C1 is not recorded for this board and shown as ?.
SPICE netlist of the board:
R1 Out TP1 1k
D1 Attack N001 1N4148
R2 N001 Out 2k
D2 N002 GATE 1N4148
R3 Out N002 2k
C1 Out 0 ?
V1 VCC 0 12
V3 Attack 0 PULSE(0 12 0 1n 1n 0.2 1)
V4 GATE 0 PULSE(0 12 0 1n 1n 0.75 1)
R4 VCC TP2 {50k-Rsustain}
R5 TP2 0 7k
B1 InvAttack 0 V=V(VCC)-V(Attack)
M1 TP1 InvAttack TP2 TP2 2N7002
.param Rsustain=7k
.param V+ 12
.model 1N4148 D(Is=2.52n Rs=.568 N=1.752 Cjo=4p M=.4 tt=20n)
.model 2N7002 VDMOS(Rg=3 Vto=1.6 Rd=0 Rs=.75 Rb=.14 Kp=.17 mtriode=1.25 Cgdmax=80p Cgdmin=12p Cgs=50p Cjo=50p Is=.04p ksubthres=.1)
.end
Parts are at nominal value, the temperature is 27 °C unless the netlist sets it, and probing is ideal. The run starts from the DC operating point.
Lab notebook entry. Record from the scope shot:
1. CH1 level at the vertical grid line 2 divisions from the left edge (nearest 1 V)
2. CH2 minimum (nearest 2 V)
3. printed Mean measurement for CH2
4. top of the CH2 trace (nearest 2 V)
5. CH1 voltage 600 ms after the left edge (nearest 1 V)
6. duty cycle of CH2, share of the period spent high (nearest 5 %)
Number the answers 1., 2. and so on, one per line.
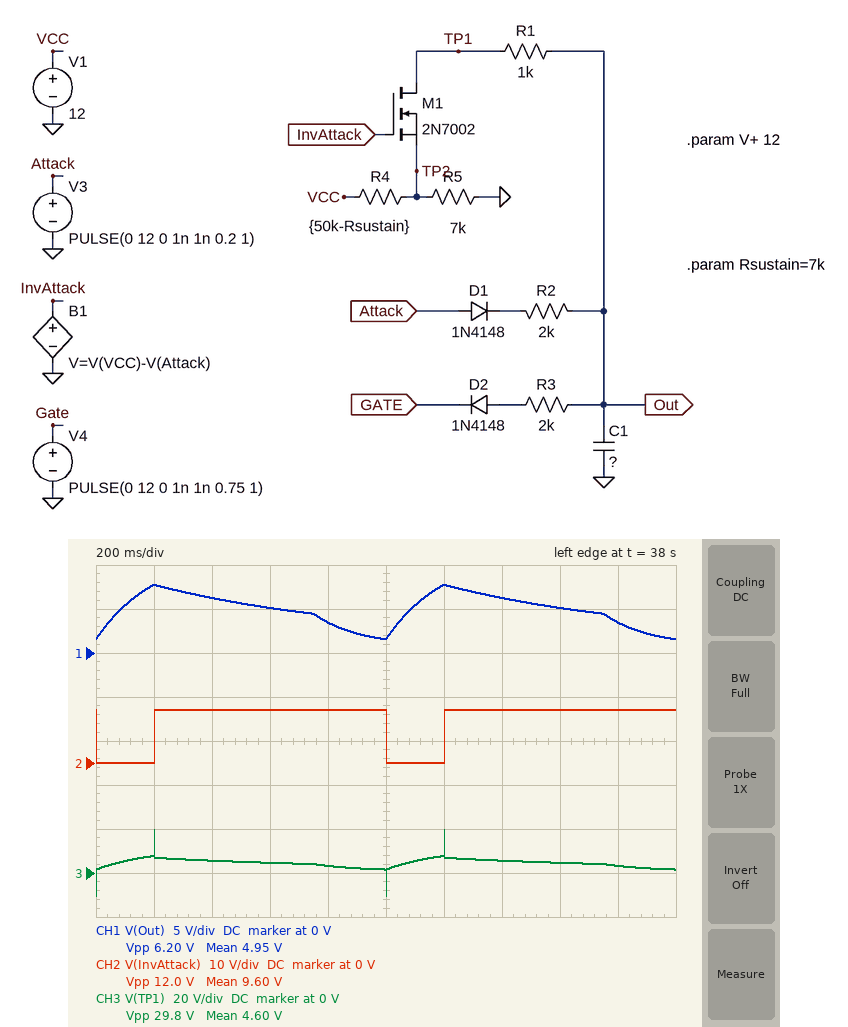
1. 6 V
2. 0 V
3. 9.60 V
4. 12 V
5. 5 V
6. 80 %
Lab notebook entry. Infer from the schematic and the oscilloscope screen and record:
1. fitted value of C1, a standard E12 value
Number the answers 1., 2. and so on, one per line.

1. 100 µF
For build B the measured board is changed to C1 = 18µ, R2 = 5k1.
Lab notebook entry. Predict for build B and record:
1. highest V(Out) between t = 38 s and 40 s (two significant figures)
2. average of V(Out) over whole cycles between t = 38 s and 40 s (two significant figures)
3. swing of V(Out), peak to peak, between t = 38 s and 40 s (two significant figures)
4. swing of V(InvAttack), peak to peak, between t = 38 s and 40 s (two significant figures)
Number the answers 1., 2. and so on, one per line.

1. 10 V
2. 3.6 V
3. 9.5 V
4. 12 V
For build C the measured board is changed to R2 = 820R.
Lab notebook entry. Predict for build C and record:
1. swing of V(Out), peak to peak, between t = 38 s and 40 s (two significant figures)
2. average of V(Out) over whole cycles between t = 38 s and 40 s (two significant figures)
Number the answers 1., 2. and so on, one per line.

1. 8.7 V
2. 6.7 V
